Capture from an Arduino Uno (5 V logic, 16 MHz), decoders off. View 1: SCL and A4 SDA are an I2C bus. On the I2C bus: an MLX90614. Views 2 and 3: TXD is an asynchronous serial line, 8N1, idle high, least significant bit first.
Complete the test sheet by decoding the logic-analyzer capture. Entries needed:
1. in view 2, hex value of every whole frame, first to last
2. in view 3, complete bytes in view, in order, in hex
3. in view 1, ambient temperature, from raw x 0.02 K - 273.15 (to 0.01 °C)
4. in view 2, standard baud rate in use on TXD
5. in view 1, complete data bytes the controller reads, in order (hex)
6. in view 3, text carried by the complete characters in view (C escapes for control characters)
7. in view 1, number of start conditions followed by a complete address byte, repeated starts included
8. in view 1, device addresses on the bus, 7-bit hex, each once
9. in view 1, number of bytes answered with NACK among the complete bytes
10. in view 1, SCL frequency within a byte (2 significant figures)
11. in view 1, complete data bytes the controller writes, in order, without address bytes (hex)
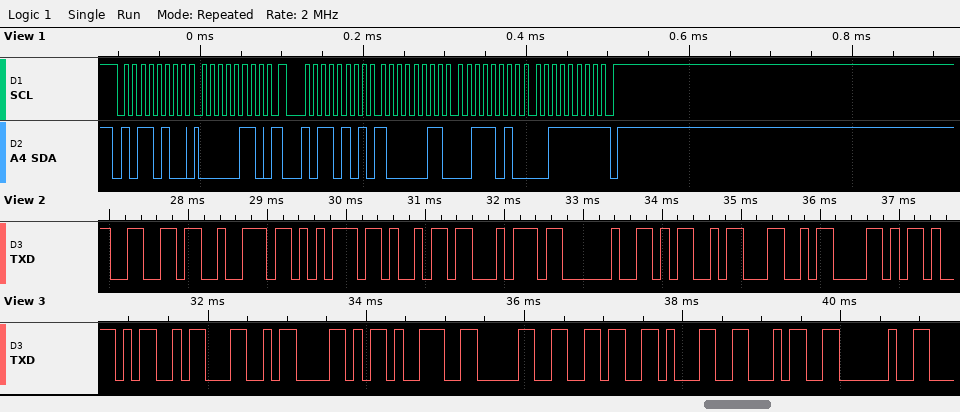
0x66 0x72 0x75 0x69 0x74 0x20 0x4D 0x4C 0x58
0x4D 0x4C 0x58 0x39 0x30 0x36 0x31 0x34 0x20
26.43 °C
9600 baud
83 3A 3F
"MLX90614 "
2
0x5A
1
100 kHz
06
